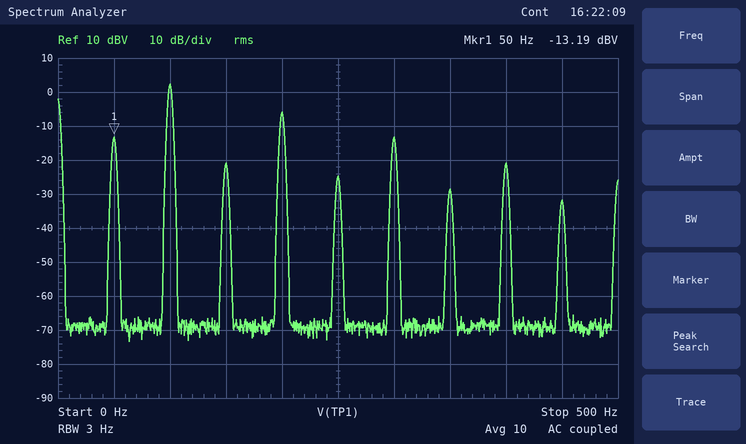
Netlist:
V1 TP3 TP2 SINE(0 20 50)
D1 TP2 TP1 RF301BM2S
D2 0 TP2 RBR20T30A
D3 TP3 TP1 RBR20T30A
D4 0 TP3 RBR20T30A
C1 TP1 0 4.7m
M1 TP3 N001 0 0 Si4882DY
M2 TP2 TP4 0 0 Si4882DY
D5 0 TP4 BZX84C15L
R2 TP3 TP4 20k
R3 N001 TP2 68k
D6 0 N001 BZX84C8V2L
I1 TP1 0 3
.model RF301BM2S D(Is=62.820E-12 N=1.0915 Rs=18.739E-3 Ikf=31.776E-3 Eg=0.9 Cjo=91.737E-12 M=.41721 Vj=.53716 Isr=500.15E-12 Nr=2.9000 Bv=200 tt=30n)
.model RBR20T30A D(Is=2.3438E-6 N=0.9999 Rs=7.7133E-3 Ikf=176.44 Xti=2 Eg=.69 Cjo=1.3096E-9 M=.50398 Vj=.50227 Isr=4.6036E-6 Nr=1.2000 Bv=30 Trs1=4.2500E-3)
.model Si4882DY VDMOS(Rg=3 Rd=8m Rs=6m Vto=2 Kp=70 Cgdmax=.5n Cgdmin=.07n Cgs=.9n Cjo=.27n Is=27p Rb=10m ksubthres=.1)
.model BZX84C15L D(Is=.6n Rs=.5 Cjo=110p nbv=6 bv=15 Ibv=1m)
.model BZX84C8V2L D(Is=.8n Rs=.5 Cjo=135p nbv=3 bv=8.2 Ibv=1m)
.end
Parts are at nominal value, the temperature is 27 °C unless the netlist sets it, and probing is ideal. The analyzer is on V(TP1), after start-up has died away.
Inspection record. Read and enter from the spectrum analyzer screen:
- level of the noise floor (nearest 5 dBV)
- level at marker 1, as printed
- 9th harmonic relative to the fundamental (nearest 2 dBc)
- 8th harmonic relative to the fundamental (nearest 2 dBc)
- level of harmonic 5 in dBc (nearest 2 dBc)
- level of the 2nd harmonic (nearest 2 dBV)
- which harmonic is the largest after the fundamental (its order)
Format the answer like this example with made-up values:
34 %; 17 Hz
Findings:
-70 dBV; -13.19 dBV; -18 dBc; -8 dBc; -12 dBc; 2 dBV; 2
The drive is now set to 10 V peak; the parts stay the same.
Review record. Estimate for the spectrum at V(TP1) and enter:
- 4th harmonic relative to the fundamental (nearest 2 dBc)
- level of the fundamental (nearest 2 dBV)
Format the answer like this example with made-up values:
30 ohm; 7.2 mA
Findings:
4 dBc; -14 dBV
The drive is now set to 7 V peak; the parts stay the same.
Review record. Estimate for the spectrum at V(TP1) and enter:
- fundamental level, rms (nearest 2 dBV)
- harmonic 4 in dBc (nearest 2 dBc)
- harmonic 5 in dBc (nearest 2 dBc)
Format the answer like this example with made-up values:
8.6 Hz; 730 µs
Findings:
-14 dBV; 2 dBc; -14 dBc
